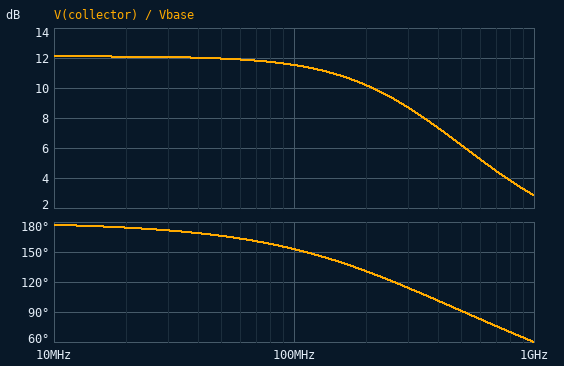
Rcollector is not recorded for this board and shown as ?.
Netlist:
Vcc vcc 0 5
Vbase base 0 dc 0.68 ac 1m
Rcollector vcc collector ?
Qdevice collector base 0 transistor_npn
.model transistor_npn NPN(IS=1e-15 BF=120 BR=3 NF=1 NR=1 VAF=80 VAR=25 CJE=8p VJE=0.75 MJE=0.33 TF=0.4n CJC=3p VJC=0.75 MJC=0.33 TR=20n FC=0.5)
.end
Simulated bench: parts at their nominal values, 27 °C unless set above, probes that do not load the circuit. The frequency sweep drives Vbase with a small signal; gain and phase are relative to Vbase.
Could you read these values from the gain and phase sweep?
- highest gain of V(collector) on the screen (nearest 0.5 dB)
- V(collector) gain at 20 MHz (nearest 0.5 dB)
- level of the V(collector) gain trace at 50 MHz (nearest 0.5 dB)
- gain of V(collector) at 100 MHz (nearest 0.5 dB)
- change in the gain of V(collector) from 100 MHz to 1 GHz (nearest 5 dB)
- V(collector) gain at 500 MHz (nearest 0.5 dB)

12.0 dB
12.0 dB
12.0 dB
11.5 dB
-10 dB
6.0 dB
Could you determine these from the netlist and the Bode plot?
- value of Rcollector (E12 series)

390 Ω
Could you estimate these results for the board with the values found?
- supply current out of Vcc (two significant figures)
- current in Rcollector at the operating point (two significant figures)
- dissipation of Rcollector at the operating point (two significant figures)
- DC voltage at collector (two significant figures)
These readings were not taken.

270 µA
270 µA
28 µW
4.9 V
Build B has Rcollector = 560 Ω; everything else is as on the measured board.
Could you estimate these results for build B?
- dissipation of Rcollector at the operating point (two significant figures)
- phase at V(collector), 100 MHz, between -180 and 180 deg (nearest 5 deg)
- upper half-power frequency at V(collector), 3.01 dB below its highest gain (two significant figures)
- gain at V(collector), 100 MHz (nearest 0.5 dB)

40 µW
145 deg
180 MHz
14.0 dB
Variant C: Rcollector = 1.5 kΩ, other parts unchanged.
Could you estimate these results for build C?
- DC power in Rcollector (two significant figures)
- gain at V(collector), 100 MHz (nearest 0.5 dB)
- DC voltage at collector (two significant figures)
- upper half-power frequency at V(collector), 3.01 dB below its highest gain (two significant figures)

110 µW
18.5 dB
4.6 V
65 MHz
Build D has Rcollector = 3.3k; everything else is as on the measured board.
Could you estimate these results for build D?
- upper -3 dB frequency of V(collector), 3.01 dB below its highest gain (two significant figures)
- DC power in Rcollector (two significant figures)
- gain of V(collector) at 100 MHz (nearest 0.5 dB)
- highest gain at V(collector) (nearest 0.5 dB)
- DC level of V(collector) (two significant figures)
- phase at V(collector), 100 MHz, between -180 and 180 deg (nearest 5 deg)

29 MHz
230 µW
19.5 dB
30.5 dB
4.1 V
100 deg
